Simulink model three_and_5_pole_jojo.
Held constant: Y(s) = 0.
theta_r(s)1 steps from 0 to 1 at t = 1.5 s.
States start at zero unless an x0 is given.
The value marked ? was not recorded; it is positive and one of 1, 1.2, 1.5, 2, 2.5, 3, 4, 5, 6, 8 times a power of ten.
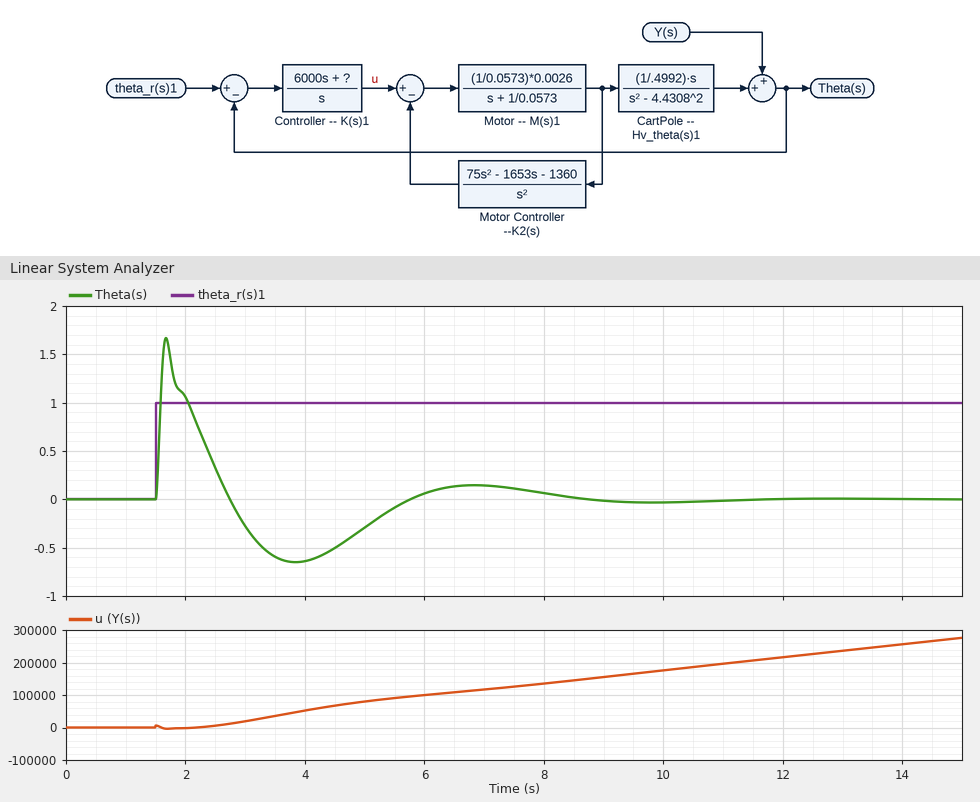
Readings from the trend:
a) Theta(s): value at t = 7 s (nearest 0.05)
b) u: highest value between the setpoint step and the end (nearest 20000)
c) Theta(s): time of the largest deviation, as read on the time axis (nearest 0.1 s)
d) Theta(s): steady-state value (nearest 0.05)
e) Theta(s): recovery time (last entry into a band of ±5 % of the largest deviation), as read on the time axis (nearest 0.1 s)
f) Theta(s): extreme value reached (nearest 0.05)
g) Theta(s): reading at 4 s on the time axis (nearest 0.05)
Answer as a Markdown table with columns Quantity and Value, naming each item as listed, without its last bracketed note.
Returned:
| Quantity | Value |
|---|---|
| Theta(s): value at t = 7 s | 0.15 |
| u: highest value between the setpoint step and the end | 280000 |
| Theta(s): time of the largest deviation, as read on the time axis | 1.7 s |
| Theta(s): steady-state value | 0.00 |
| Theta(s): recovery time (last entry into a band of ±5 % of the largest deviation), as read on the time axis | 7.8 s |
| Theta(s): extreme value reached | 1.65 |
| Theta(s): reading at 4 s on the time axis | -0.65 |
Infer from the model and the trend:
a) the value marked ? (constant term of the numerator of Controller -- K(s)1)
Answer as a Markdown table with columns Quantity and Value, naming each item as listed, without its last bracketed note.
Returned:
| Quantity | Value |
|---|---|
| the value marked ? (constant term of the numerator of Controller -- K(s)1) | 20000 |
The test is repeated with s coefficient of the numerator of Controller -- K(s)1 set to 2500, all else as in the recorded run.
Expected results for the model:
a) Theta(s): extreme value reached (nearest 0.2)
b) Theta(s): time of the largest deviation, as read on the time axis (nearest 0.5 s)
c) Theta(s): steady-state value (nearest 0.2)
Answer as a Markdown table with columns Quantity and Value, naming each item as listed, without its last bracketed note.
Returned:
| Quantity | Value |
|---|---|
| Theta(s): extreme value reached | 2.4 |
| Theta(s): time of the largest deviation, as read on the time axis | 2.0 s |
| Theta(s): steady-state value | 0.0 |
